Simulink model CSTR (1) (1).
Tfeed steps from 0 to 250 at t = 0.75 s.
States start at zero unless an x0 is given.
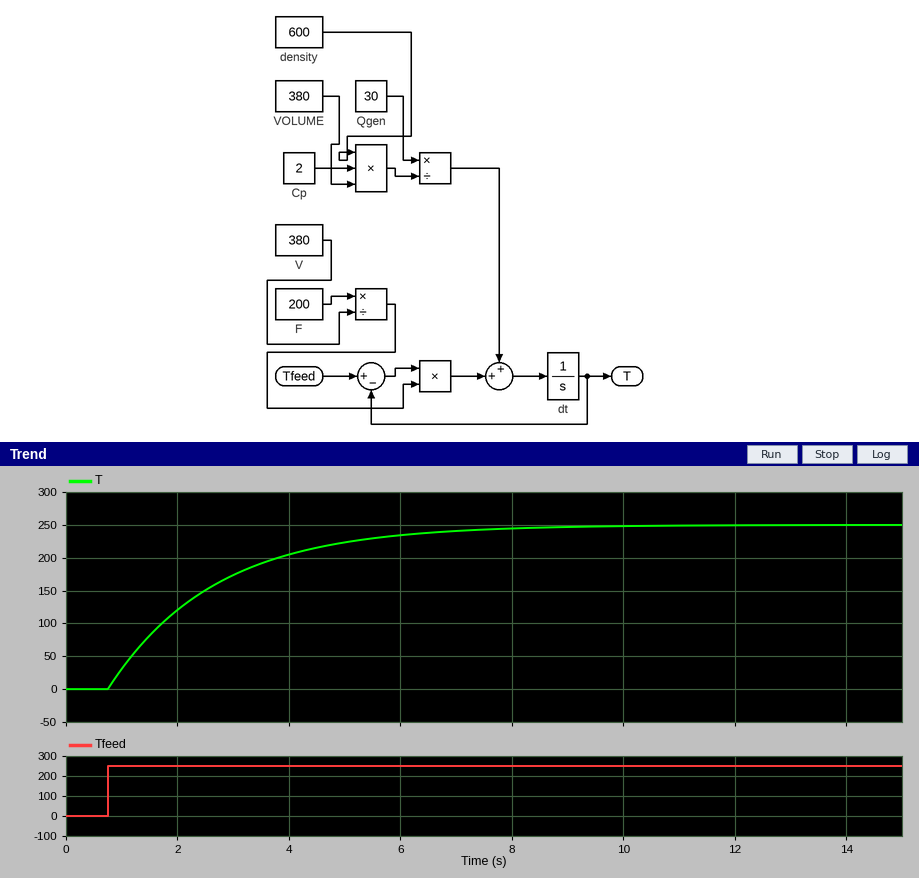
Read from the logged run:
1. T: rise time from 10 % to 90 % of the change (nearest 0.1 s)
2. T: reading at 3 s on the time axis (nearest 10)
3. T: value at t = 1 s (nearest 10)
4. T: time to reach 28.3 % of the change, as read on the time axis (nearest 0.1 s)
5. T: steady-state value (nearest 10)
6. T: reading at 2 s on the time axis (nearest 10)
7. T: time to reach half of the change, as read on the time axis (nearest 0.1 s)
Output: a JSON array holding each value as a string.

["4.2 s", "170", "30", "1.4 s", "250", "120", "2.1 s"]
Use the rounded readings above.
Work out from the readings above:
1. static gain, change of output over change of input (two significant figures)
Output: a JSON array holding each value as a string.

["1.0"]
